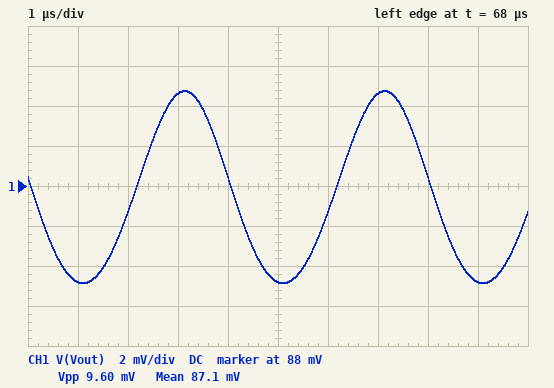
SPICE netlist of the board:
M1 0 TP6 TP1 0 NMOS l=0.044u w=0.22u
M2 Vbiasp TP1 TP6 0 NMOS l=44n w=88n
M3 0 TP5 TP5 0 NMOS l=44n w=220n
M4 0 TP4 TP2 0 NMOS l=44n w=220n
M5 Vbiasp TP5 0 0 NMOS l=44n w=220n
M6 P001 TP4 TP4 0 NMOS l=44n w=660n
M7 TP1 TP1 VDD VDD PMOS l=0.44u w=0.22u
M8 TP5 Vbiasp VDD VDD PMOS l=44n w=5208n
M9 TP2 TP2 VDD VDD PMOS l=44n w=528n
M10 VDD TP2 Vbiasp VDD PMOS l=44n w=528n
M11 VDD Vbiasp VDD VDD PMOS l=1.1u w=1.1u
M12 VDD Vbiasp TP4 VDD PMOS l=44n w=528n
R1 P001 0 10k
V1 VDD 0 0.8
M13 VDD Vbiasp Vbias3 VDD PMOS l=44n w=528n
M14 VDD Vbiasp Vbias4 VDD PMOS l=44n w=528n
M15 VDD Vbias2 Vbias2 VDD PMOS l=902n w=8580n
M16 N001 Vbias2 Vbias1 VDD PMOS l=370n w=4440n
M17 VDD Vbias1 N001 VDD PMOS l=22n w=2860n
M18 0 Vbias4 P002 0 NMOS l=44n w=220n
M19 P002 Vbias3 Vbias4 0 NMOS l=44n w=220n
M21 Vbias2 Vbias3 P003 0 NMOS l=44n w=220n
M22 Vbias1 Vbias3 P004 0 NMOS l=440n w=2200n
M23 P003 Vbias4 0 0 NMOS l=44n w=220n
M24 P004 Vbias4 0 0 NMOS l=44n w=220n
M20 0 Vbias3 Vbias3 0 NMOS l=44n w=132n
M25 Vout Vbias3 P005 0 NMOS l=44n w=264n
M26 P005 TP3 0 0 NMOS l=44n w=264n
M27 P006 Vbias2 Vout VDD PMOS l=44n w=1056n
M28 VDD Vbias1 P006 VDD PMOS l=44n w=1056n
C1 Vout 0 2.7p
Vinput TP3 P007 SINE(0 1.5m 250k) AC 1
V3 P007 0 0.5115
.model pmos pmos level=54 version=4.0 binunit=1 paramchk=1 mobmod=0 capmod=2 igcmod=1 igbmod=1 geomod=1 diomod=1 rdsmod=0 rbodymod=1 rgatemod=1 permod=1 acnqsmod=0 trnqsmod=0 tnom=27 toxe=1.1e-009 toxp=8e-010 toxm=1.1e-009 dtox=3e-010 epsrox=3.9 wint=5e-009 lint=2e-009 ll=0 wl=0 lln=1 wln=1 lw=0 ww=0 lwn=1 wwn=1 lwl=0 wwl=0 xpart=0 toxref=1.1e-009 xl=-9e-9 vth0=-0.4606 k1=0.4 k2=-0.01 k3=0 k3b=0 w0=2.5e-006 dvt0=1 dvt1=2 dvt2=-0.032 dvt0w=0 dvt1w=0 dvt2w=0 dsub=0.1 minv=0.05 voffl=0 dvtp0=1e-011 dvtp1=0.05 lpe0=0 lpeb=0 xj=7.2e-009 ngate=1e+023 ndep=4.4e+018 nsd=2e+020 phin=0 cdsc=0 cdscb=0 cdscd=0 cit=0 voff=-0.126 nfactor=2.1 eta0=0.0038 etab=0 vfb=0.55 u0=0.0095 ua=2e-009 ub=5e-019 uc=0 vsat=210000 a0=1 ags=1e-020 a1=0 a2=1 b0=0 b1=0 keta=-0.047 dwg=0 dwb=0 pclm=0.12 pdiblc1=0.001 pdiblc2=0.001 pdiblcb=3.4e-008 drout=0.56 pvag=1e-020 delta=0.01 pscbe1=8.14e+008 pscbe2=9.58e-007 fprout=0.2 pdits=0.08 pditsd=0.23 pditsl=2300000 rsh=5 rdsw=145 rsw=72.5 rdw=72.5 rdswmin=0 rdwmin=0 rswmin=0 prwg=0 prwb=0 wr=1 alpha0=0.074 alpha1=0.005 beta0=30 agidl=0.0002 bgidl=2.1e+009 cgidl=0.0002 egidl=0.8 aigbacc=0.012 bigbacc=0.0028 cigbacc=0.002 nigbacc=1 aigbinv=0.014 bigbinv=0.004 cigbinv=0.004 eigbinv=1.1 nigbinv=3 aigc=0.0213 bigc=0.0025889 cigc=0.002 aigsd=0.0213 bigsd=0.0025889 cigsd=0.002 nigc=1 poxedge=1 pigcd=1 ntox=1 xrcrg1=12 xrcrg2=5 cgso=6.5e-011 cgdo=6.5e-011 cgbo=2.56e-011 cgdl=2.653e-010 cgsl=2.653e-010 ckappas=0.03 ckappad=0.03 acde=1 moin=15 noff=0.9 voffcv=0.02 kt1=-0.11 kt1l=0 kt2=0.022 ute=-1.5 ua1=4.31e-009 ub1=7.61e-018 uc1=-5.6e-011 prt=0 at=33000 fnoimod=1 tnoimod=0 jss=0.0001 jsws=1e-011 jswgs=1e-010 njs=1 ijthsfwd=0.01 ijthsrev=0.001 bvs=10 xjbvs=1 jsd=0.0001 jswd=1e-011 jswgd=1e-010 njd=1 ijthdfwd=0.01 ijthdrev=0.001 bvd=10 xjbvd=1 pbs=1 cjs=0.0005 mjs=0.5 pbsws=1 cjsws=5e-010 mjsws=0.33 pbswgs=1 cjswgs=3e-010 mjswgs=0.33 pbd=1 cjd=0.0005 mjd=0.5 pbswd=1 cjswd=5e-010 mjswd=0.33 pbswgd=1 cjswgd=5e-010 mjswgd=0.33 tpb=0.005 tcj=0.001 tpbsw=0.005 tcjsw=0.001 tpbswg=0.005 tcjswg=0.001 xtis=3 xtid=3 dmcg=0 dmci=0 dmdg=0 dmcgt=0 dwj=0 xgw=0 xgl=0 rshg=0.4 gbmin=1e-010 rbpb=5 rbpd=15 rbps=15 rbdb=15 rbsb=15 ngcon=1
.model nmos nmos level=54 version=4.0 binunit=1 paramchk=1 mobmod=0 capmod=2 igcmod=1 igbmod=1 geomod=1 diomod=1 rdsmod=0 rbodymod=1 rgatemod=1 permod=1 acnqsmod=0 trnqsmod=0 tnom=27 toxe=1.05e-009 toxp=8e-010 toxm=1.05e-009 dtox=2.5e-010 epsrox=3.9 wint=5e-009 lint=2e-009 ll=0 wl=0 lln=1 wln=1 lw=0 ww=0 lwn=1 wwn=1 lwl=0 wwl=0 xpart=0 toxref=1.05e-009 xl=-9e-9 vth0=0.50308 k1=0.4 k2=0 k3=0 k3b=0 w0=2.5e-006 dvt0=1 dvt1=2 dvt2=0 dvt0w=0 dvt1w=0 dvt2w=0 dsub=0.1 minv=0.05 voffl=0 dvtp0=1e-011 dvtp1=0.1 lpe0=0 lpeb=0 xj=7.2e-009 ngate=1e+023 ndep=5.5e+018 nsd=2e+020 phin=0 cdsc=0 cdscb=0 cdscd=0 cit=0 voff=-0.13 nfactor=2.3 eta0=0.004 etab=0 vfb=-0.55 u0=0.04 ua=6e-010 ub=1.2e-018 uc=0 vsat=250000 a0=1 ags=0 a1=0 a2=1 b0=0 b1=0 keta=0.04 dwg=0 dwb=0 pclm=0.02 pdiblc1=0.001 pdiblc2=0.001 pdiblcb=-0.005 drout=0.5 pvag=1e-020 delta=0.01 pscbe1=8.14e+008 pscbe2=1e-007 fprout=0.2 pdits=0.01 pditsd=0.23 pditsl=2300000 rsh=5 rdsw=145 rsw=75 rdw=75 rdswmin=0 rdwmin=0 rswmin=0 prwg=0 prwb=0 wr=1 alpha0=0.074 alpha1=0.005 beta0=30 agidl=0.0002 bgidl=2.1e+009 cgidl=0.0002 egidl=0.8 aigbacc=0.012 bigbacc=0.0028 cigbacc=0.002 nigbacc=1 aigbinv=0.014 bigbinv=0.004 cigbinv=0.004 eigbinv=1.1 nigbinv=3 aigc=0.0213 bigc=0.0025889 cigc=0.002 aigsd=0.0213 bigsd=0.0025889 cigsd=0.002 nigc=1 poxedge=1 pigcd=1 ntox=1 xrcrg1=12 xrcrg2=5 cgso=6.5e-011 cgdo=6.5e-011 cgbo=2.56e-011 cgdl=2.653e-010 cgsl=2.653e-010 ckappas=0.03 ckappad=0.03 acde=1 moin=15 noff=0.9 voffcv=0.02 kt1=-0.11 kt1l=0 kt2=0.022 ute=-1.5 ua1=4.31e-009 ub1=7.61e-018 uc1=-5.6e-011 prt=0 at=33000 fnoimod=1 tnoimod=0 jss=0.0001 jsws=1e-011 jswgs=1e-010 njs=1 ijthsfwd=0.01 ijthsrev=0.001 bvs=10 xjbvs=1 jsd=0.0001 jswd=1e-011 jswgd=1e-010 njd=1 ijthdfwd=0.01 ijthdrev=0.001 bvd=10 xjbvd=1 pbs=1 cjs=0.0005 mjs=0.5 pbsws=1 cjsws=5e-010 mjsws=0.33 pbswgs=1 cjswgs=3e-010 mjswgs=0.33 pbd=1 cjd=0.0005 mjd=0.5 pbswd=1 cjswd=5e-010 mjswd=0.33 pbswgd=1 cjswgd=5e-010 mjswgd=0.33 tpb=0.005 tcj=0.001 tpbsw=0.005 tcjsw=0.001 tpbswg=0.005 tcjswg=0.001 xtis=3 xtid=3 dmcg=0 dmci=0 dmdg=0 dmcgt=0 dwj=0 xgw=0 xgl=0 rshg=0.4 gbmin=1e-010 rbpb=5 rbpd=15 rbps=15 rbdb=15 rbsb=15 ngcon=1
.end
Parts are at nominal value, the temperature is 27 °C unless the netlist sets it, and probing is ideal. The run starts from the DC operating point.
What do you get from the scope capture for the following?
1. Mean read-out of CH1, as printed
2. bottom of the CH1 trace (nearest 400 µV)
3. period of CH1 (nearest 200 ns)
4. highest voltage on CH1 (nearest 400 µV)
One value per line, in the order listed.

87.1 mV
83.2 mV
4.0 µs
92.8 mV
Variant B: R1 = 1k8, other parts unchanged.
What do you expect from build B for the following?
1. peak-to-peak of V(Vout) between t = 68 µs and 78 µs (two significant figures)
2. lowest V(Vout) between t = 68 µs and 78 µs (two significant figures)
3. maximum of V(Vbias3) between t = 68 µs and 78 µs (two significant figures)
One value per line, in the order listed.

7.1 mV
720 mV
690 mV
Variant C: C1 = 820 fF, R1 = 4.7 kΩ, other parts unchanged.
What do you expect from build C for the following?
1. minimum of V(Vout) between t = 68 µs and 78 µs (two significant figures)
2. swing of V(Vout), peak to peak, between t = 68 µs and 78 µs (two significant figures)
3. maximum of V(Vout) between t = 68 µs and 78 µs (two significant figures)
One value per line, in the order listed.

370 mV
220 mV
590 mV
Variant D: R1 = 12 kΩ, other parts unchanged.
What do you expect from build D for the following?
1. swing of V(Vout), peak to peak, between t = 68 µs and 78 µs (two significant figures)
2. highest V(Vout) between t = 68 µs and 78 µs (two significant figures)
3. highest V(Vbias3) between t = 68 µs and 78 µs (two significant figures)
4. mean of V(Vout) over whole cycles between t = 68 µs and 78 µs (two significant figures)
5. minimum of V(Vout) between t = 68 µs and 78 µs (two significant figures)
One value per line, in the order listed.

7.8 mV
85 mV
680 mV
81 mV
78 mV
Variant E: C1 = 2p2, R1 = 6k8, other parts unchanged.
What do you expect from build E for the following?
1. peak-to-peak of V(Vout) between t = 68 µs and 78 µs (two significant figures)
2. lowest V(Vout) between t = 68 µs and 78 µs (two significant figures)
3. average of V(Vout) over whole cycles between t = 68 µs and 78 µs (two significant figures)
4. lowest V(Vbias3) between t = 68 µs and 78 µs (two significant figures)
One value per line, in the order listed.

22 mV
100 mV
110 mV
680 mV
